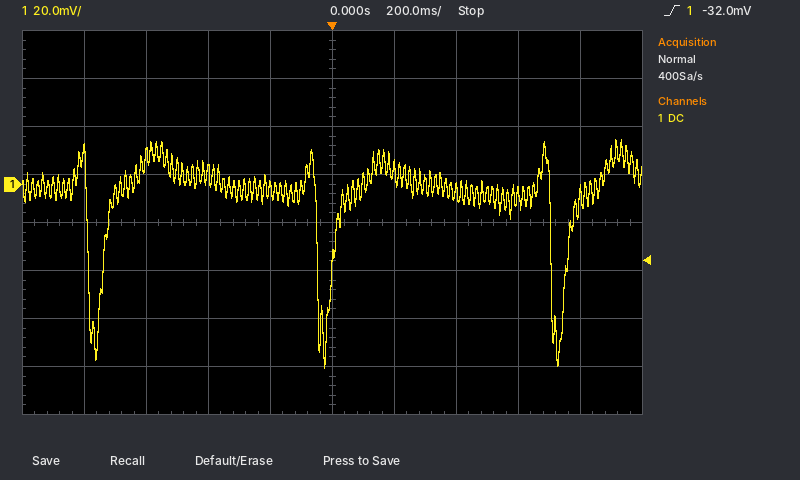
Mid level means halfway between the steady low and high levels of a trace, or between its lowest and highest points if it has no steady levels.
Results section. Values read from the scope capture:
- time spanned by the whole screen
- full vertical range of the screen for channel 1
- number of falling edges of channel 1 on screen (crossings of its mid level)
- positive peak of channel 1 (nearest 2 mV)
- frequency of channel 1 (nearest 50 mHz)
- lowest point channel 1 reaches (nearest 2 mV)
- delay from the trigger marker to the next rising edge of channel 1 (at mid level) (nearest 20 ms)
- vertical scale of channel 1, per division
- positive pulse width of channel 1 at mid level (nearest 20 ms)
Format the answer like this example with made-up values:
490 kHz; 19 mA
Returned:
2 s; 160 mV; 3; 18 mV; 1.35 Hz; -76 mV; 760 ms; 20 mV; 700 ms
